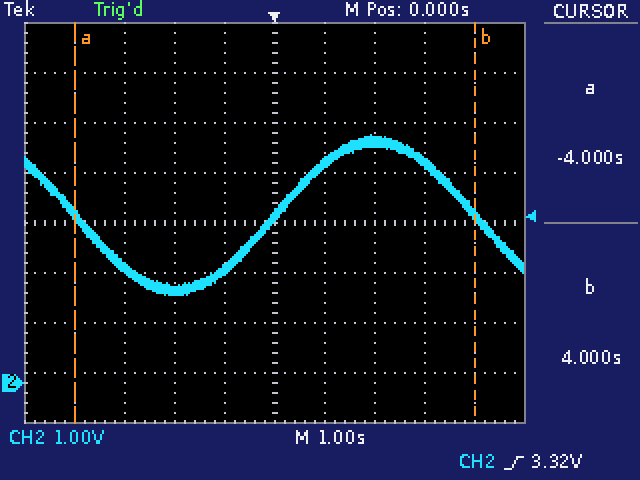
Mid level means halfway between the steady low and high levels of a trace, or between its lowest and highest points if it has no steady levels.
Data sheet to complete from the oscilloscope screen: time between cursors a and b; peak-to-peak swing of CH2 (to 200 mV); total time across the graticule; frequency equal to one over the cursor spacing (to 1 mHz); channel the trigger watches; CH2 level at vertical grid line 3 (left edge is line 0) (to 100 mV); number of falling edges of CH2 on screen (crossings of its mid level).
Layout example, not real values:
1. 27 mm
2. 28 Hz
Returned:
1. 8.0 s
2. 3.2 V
3. 10 s
4. 125 mHz
5. CH2
6. 1.8 V
7. 2
